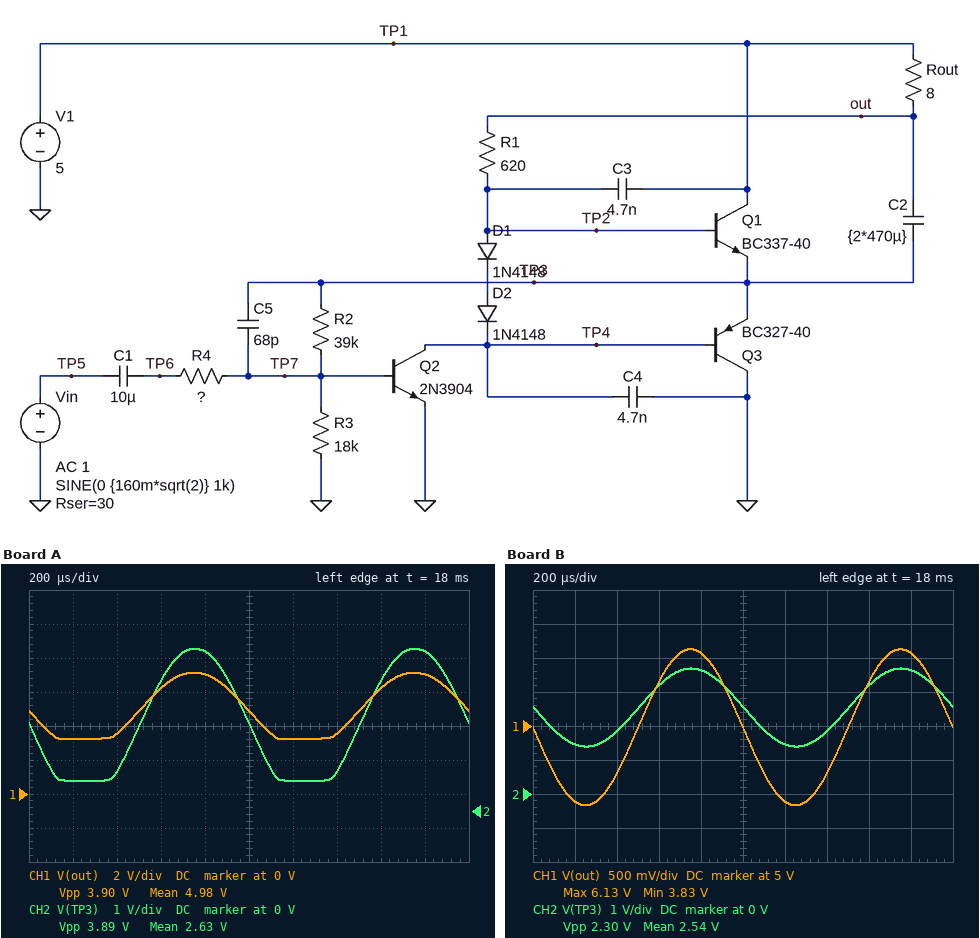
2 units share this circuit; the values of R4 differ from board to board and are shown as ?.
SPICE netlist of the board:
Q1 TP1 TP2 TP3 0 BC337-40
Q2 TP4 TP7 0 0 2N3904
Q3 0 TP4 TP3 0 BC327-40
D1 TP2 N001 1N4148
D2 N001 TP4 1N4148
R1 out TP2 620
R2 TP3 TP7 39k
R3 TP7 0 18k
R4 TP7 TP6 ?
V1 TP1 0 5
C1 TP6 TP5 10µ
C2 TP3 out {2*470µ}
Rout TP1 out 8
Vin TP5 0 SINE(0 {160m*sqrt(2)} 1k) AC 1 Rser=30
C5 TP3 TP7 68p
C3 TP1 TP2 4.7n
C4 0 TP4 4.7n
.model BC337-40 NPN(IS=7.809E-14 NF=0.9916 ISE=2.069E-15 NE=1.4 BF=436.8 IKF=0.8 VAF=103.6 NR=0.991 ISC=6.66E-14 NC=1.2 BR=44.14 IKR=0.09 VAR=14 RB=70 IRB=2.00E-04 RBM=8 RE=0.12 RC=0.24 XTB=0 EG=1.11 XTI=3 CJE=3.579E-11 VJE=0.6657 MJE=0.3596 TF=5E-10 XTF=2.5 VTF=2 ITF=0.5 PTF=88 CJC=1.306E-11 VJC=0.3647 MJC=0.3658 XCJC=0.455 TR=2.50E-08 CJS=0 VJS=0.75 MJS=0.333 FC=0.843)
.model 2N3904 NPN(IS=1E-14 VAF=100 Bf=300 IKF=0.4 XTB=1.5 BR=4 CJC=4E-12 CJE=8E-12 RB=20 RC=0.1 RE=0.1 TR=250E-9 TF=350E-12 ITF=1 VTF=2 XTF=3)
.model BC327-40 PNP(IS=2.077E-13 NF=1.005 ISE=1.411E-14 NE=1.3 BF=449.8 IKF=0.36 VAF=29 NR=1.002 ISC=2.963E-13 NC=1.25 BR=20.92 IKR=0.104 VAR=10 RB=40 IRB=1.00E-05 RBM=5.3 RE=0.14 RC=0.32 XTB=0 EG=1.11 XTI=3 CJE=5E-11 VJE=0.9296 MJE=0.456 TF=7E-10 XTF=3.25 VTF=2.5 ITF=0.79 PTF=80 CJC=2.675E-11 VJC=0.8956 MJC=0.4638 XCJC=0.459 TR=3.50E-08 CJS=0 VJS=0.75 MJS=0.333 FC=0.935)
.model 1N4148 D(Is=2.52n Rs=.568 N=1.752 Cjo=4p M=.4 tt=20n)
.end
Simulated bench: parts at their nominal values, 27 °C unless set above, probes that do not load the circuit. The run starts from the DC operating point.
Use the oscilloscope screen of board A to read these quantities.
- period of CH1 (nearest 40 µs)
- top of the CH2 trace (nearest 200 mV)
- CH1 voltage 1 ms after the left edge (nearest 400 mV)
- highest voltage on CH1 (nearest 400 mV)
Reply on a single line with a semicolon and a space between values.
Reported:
1.00 ms; 4.8 V; 4.8 V; 7.2 V
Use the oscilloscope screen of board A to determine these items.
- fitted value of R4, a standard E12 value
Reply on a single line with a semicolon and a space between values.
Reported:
3.3 kΩ
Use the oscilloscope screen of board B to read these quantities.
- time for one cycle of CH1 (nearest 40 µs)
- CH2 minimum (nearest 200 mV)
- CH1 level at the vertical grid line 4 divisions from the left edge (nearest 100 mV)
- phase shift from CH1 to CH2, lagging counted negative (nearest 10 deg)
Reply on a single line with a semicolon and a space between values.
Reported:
1.00 ms; 1.4 V; 6.1 V; 0 deg
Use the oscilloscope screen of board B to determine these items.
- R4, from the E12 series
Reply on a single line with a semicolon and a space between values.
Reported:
6.8 kΩ
